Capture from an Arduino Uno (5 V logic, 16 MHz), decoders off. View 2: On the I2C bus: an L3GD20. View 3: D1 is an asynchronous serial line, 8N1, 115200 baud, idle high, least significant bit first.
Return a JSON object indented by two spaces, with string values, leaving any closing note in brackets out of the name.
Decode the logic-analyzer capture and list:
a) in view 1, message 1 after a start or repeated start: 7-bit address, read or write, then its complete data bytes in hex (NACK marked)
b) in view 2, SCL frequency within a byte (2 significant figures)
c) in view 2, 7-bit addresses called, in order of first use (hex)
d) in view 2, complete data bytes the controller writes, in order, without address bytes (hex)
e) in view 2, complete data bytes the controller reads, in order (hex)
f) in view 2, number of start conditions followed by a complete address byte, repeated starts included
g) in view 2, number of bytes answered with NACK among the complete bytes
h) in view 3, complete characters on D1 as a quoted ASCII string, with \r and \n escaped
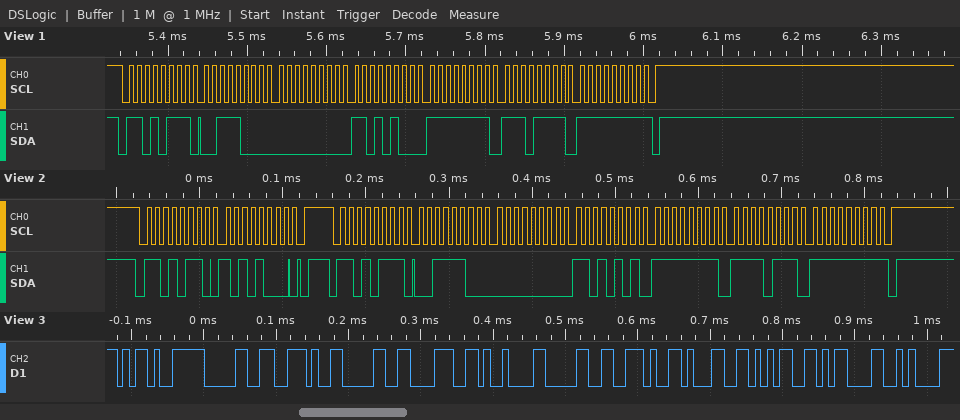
{
  "in view 1, message 1 after a start or repeated start: 7-bit address, read or write, then its complete data bytes in hex": "0x6B read: 38 00 D4 FF EF FF NACK",
  "in view 2, SCL frequency within a byte": "100 kHz",
  "in view 2, 7-bit addresses called, in order of first use": "0x6B",
  "in view 2, complete data bytes the controller writes, in order, without address bytes": "A8",
  "in view 2, complete data bytes the controller reads, in order": "3C 00 D5 FF F7 FF",
  "in view 2, number of start conditions followed by a complete address byte, repeated starts included": "2",
  "in view 2, number of bytes answered with NACK among the complete bytes": "1",
  "in view 3, complete characters on D1 as a quoted ASCII string, with \\r and \\n escaped": "\"-0.08\\t0.15\\r\\n\""
}
